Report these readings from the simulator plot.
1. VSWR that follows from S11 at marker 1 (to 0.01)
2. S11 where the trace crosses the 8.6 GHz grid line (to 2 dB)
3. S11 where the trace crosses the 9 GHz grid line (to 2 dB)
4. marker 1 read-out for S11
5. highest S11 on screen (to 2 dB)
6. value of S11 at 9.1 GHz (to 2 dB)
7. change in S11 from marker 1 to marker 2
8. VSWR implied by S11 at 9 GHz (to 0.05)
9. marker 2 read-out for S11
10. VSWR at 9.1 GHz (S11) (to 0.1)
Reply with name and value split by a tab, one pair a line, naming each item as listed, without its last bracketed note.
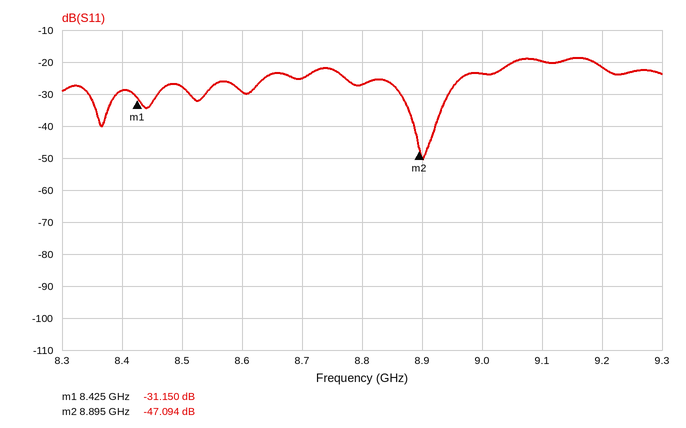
VSWR that follows from S11 at marker 1	1.06
S11 where the trace crosses the 8.6 GHz grid line	-30 dB
S11 where the trace crosses the 9 GHz grid line	-24 dB
marker 1 read-out for S11	-31.150 dB
highest S11 on screen	-18 dB
value of S11 at 9.1 GHz	-20 dB
change in S11 from marker 1 to marker 2	-15.944 dB
VSWR implied by S11 at 9 GHz	1.15
marker 2 read-out for S11	-47.094 dB
VSWR at 9.1 GHz (S11)	1.2
